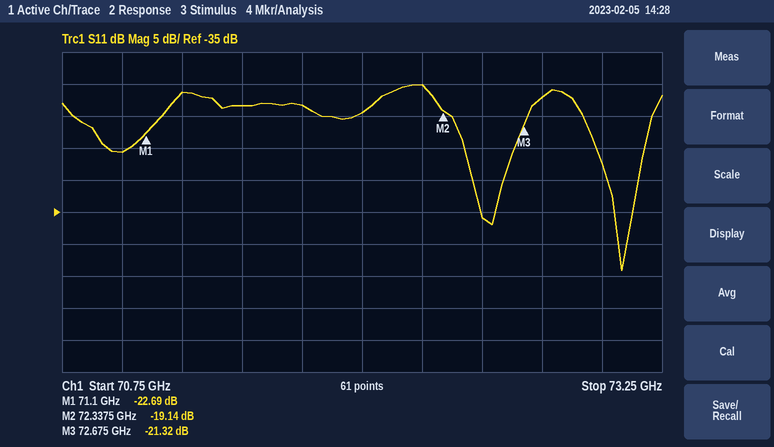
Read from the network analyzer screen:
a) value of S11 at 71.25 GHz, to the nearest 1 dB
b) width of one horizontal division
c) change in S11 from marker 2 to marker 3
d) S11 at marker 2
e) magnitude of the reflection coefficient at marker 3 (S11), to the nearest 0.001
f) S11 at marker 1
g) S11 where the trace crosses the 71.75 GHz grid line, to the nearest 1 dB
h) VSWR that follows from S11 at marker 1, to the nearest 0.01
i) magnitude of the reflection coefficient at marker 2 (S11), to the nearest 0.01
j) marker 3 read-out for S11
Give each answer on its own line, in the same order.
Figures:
-16 dB
250 MHz
-2.18 dB
-19.14 dB
0.086
-22.69 dB
-18 dB
1.16
0.11
-21.32 dB
